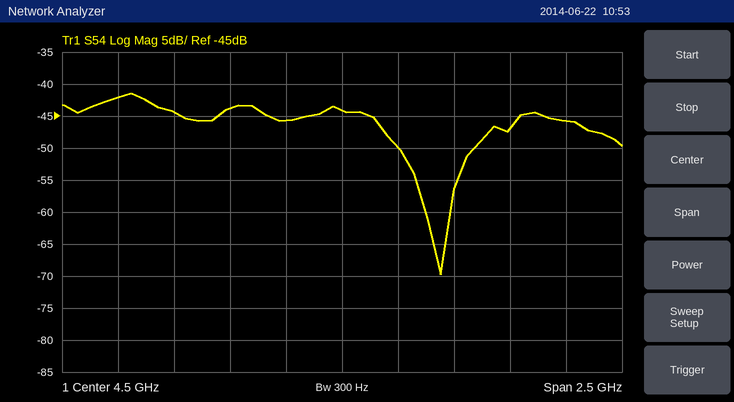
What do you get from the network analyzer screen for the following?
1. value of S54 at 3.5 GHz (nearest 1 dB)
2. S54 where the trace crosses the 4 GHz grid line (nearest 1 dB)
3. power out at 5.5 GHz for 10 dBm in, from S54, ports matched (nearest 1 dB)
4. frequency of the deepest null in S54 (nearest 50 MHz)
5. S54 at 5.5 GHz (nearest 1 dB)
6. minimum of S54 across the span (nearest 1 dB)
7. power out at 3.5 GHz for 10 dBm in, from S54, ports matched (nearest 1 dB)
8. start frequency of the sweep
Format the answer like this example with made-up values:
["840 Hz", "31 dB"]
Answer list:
["-42 dB", "-44 dB", "-36 dBm", "4.95 GHz", "-46 dB", "-70 dB", "-32 dBm", "3.25 GHz"]
